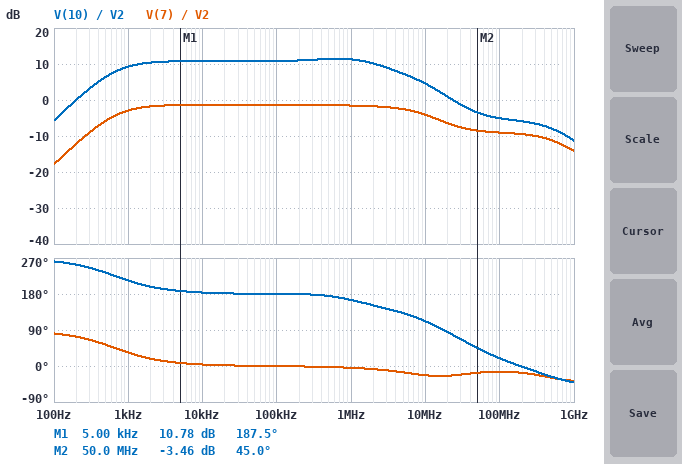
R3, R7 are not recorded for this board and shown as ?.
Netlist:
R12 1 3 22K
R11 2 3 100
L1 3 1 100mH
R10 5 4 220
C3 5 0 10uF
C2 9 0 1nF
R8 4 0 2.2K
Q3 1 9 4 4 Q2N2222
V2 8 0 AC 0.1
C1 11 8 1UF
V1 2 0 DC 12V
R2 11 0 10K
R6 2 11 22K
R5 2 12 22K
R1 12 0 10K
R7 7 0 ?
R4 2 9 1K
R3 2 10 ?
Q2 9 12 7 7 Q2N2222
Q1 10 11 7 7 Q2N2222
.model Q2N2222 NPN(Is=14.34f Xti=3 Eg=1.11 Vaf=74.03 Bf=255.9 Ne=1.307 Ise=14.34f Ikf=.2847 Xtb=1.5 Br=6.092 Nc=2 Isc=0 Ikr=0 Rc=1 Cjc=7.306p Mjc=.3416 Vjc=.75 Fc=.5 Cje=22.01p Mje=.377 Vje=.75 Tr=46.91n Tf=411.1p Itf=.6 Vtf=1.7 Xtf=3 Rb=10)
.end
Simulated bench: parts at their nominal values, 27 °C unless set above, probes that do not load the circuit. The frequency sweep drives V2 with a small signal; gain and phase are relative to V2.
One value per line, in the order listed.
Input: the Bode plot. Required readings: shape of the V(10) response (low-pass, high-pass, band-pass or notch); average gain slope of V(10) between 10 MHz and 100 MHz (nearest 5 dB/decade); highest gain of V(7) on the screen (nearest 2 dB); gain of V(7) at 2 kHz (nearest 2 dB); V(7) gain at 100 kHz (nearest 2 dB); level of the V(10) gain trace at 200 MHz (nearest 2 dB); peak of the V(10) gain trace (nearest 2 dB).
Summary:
band-pass
-10 dB/decade
-2 dB
-2 dB
-2 dB
-6 dB
12 dB
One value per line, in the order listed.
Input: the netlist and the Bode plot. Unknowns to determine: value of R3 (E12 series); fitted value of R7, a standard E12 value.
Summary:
1.2 kΩ
150 Ω
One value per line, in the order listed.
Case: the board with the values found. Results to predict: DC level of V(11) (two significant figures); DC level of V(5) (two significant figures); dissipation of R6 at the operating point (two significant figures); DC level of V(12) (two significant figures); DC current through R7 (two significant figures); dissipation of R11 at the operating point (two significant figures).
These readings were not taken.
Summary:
3.3 V
2.1 V
3.5 mW
3.3 V
17 mA
87 µW
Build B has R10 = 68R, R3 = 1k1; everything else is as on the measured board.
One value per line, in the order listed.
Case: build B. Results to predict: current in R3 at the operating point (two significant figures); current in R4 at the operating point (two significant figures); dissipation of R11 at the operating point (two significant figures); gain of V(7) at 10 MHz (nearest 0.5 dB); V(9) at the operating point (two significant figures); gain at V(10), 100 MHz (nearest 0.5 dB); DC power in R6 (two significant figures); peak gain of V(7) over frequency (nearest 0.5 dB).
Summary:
8.4 mA
9.2 mA
96 µW
-4.0 dB
2.8 V
-2.0 dB
3.4 mW
-1.0 dB
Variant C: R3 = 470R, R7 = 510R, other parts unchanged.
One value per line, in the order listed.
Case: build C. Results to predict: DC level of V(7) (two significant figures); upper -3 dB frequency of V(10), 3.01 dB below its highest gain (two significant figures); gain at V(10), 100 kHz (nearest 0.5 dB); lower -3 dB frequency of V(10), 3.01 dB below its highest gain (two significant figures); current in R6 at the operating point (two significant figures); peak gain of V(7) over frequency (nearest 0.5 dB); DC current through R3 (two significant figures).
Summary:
3.0 V
1.1 MHz
18.0 dB
39 Hz
380 µA
-0.5 dB
2.9 mA
